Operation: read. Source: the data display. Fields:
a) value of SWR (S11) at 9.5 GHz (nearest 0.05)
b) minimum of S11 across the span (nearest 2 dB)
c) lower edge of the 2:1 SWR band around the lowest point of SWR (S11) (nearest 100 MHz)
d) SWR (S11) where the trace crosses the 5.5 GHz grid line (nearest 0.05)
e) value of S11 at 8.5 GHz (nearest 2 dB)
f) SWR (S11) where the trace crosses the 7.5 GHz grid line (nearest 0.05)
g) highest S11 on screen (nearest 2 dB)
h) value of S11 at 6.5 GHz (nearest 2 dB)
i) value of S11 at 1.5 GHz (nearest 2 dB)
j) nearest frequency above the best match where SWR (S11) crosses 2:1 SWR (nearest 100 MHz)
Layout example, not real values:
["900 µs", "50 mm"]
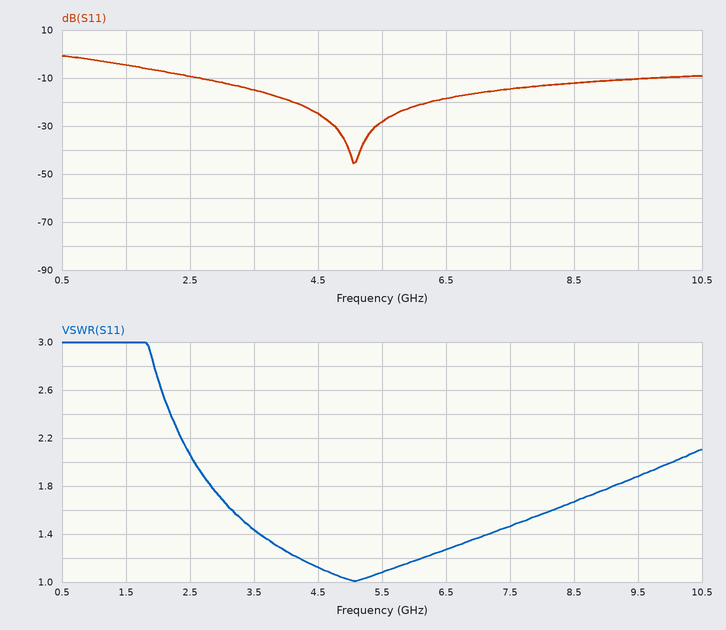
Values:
["1.90", "-46 dB", "2.6 GHz", "1.10", "-12 dB", "1.45", "0 dB", "-18 dB", "-4 dB", "10.0 GHz"]
